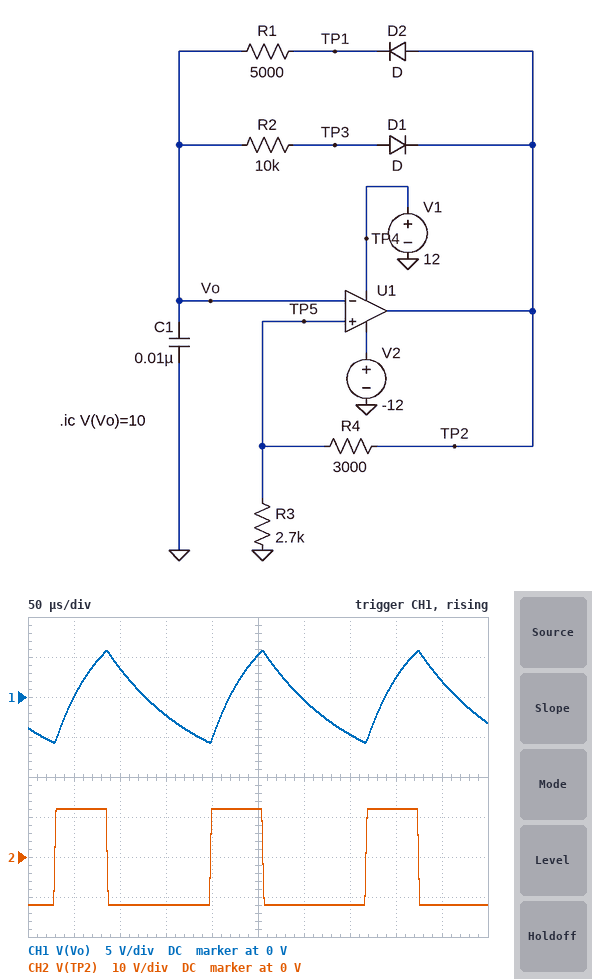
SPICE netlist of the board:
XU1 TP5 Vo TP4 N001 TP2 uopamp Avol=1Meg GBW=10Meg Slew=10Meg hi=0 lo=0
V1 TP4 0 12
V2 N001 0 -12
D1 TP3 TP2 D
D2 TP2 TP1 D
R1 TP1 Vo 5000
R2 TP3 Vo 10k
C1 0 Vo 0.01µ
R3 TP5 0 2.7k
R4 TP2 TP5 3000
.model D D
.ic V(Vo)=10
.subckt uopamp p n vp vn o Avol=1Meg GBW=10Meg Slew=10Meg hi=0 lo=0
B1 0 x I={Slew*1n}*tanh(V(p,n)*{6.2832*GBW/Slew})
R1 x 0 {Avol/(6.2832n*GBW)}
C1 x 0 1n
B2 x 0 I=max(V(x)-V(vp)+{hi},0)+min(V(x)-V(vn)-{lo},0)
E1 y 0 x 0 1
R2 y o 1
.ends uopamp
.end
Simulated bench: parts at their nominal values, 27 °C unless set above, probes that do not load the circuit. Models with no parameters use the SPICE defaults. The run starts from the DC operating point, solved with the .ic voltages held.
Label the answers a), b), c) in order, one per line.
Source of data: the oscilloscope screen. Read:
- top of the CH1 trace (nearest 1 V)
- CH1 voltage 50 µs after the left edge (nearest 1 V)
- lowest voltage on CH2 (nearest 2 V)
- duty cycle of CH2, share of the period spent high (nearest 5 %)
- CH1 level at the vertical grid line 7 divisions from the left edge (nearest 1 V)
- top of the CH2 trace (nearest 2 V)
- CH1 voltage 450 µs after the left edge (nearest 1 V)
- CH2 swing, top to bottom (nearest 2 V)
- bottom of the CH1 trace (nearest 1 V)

a) 6 V
b) 0 V
c) -12 V
d) 35 %
e) -5 V
f) 12 V
g) 2 V
h) 24 V
i) -6 V
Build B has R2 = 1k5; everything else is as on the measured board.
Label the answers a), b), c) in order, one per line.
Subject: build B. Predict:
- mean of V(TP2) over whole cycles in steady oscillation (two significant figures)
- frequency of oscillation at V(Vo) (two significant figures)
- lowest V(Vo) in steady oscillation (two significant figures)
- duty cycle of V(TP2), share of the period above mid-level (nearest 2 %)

a) 6.2 V
b) 13 kHz
c) -5.8 V
d) 76 %
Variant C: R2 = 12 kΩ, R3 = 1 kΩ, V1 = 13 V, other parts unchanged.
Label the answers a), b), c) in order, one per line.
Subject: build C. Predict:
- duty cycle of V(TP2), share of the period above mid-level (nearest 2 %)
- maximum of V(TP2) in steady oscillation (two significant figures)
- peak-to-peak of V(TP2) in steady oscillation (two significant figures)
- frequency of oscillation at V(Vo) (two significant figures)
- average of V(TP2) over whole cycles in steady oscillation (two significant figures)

a) 28 %
b) 13 V
c) 25 V
d) 10 kHz
e) -4.8 V
